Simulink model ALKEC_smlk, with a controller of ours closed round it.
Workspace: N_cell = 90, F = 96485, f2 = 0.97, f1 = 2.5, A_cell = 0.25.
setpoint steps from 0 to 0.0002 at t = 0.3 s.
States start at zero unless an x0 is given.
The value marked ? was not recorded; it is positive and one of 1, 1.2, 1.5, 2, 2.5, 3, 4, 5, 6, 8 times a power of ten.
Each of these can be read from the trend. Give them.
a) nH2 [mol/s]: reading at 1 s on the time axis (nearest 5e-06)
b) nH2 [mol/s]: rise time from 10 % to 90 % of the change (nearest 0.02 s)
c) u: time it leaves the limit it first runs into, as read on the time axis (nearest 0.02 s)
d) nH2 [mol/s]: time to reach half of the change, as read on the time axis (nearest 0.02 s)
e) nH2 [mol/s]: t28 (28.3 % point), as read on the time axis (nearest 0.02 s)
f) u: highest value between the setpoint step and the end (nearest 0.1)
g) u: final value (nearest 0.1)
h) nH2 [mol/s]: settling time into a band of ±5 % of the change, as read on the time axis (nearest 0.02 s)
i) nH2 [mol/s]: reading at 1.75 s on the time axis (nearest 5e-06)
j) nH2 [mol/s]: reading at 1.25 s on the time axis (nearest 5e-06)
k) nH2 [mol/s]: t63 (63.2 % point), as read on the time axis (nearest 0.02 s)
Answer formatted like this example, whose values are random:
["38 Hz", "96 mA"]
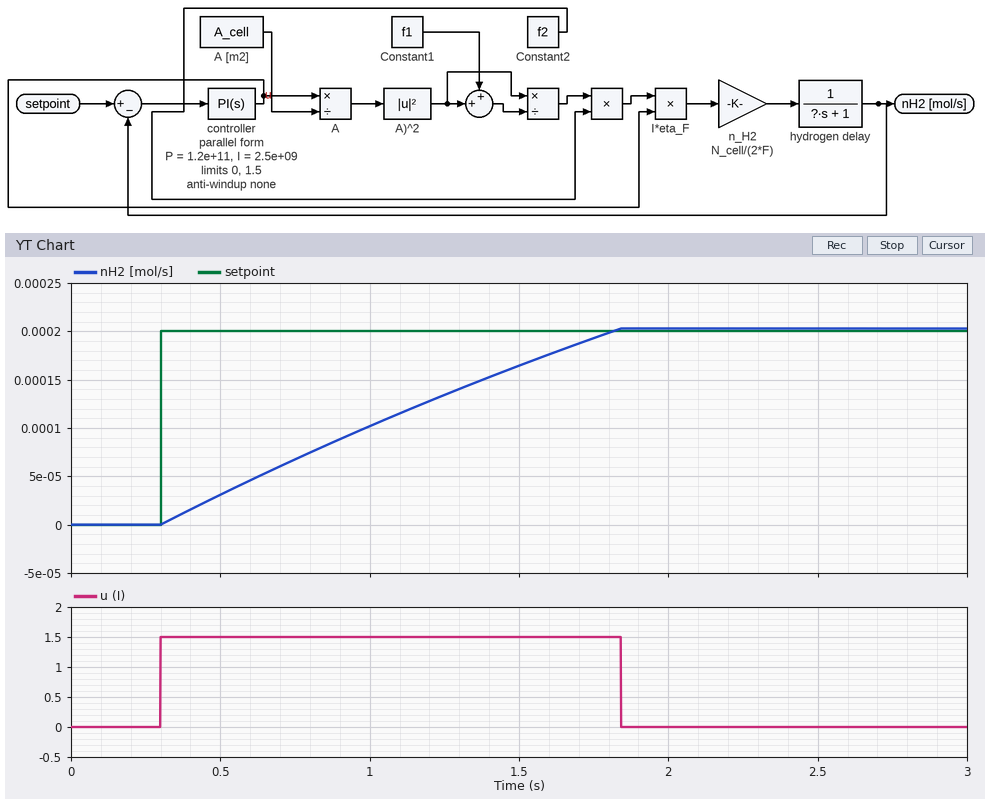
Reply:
["0.000100", "1.22 s", "1.84 s", "1.00 s", "0.68 s", "1.5", "0.0", "1.74 s", "0.000195", "0.000135", "1.20 s"]
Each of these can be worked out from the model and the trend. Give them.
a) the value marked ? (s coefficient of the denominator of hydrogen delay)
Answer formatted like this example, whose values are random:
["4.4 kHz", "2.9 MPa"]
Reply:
["4"]
